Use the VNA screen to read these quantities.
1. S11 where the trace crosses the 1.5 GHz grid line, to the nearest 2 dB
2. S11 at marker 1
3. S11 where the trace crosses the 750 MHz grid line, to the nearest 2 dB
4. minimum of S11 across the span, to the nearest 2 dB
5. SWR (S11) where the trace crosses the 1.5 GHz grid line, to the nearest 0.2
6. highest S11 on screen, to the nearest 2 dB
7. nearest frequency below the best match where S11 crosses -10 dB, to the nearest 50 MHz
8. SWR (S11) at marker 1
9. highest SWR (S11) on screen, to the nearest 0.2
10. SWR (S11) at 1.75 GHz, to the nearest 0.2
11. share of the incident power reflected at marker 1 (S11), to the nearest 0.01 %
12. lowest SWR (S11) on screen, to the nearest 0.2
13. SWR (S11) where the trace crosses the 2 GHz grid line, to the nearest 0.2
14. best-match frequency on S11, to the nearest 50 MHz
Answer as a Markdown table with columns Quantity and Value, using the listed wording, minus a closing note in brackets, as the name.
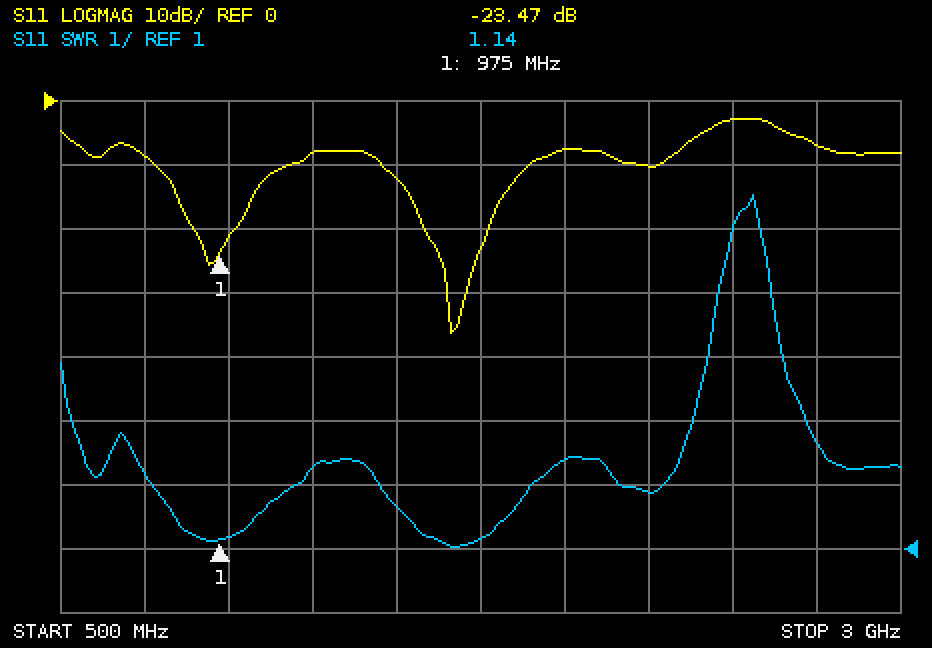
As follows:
| Quantity | Value |
|---|---|
| S11 where the trace crosses the 1.5 GHz grid line, to the nearest 2 dB | -12 dB |
| S11 at marker 1 | -23.47 dB |
| S11 where the trace crosses the 750 MHz grid line, to the nearest 2 dB | -8 dB |
| minimum of S11 across the span, to the nearest 2 dB | -36 dB |
| SWR (S11) where the trace crosses the 1.5 GHz grid line, to the nearest 0.2 | 1.6 |
| highest S11 on screen, to the nearest 2 dB | -2 dB |
| nearest frequency below the best match where S11 crosses -10 dB, to the nearest 50 MHz | 1.45 GHz |
| SWR (S11) at marker 1 | 1.14 |
| highest SWR (S11) on screen, to the nearest 0.2 | 6.6 |
| SWR (S11) at 1.75 GHz, to the nearest 0.2 | 1.2 |
| share of the incident power reflected at marker 1 (S11), to the nearest 0.01 % | 0.45 % |
| lowest SWR (S11) on screen, to the nearest 0.2 | 1.0 |
| SWR (S11) where the trace crosses the 2 GHz grid line, to the nearest 0.2 | 2.4 |
| best-match frequency on S11, to the nearest 50 MHz | 1.65 GHz |
